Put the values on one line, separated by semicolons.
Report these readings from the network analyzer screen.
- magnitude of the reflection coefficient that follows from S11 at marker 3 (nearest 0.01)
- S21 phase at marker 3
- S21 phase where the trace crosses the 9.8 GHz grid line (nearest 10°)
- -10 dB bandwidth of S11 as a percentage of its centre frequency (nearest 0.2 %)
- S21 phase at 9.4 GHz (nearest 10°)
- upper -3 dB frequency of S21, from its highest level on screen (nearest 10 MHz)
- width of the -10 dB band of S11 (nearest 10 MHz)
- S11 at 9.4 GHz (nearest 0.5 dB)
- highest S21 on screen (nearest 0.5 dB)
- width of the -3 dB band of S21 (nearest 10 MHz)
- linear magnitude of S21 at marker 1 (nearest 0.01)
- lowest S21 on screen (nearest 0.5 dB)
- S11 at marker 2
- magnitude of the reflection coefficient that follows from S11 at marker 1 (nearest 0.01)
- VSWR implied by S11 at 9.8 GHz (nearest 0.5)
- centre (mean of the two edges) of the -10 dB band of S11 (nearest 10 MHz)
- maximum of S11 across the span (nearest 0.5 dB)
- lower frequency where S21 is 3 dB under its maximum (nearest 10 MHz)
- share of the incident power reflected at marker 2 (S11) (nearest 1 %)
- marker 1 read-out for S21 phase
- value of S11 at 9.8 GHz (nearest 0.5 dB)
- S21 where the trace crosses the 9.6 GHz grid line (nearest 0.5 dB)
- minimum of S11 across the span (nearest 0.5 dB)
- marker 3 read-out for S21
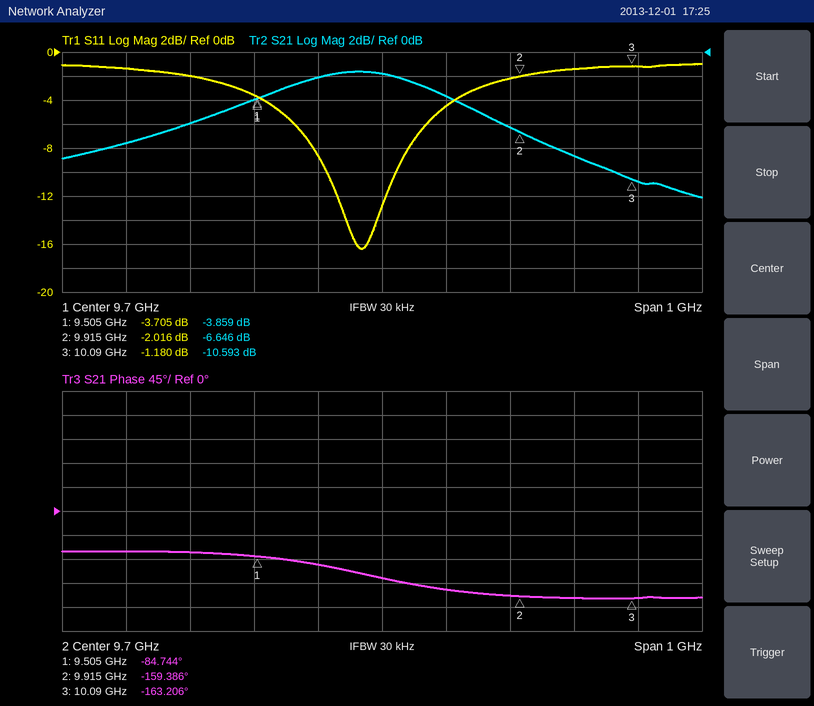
0.87; -163.206°; -150°; 1.2 %; -80°; 9.84 GHz; 110 MHz; -2.0 dB; -1.5 dB; 370 MHz; 0.64; -12.0 dB; -2.016 dB; 0.65; 4.0; 9.67 GHz; -1.0 dB; 9.47 GHz; 63 %; -84.744°; -4.5 dB; -2.0 dB; -16.5 dB; -10.593 dB
